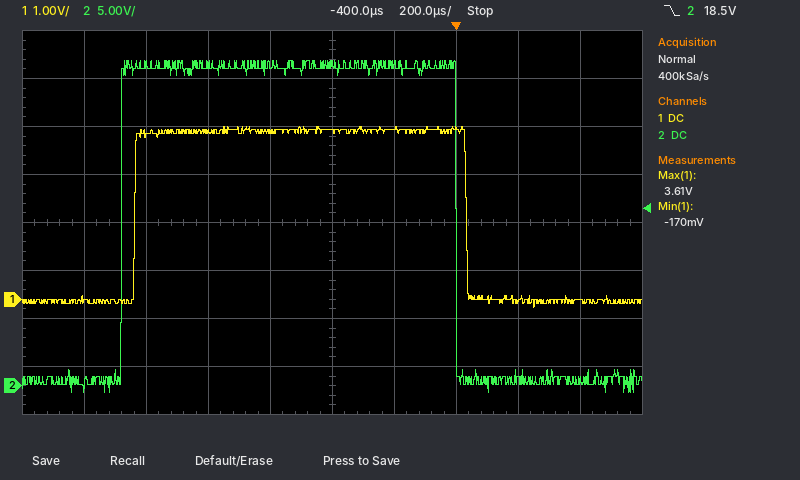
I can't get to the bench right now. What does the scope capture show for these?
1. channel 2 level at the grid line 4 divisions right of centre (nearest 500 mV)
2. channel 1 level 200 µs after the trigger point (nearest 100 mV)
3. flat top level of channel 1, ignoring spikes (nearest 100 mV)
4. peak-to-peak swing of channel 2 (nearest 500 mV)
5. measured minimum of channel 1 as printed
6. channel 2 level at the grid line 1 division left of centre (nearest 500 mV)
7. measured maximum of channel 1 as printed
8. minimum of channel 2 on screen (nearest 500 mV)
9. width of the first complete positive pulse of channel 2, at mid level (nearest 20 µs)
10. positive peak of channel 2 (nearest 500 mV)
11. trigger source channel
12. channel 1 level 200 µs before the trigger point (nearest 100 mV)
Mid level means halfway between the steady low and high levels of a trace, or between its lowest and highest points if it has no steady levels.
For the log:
500 mV
0.0 V
3.5 V
34.5 V
-170 mV
33.5 V
3.61 V
-500 mV
1.08 ms
34.0 V
channel 2
3.6 V
